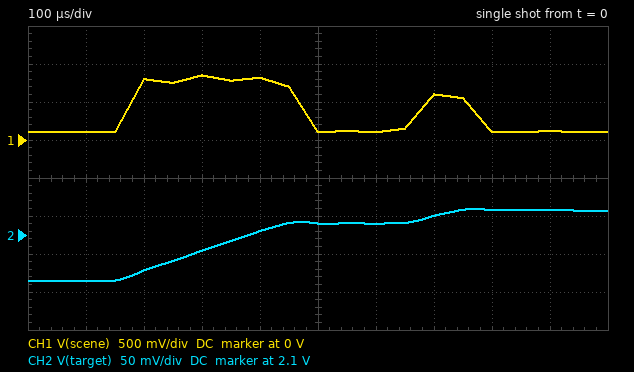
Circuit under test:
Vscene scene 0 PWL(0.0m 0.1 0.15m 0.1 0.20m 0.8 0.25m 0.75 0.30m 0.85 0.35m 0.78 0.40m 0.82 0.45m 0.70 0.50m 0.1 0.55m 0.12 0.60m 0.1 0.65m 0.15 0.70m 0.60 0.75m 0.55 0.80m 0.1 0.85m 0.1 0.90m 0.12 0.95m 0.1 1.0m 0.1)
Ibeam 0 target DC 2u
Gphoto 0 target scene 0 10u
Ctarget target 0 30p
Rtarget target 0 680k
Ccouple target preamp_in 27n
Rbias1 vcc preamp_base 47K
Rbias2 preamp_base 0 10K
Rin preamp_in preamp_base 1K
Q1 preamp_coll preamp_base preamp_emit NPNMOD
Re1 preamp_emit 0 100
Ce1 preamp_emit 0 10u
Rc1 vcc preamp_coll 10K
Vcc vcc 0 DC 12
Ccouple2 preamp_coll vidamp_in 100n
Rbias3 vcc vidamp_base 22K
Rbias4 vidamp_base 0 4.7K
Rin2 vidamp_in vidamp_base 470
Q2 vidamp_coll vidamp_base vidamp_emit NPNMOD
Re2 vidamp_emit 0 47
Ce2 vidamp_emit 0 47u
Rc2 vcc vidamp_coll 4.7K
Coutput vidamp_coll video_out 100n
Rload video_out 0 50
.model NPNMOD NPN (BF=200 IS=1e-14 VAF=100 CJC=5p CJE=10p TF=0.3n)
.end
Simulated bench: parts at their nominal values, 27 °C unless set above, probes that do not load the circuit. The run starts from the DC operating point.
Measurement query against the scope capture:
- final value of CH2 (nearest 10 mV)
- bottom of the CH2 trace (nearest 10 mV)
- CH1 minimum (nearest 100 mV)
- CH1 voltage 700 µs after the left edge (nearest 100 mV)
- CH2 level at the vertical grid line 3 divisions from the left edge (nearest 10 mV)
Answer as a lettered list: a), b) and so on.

a) 2.13 V
b) 2.04 V
c) 100 mV
d) 600 mV
e) 2.08 V
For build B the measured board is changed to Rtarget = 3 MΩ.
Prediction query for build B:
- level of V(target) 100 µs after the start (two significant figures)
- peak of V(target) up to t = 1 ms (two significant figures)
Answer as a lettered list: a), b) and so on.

a) 9.0 V
b) 9.1 V
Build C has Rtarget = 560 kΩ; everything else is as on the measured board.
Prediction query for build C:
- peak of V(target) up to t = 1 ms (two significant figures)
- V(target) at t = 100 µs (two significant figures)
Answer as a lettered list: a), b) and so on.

a) 1.8 V
b) 1.7 V
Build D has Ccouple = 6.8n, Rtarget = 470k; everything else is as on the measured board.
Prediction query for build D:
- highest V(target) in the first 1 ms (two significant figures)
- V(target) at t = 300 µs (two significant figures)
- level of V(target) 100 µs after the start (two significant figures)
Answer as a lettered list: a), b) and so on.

a) 1.7 V
b) 1.5 V
c) 1.4 V
